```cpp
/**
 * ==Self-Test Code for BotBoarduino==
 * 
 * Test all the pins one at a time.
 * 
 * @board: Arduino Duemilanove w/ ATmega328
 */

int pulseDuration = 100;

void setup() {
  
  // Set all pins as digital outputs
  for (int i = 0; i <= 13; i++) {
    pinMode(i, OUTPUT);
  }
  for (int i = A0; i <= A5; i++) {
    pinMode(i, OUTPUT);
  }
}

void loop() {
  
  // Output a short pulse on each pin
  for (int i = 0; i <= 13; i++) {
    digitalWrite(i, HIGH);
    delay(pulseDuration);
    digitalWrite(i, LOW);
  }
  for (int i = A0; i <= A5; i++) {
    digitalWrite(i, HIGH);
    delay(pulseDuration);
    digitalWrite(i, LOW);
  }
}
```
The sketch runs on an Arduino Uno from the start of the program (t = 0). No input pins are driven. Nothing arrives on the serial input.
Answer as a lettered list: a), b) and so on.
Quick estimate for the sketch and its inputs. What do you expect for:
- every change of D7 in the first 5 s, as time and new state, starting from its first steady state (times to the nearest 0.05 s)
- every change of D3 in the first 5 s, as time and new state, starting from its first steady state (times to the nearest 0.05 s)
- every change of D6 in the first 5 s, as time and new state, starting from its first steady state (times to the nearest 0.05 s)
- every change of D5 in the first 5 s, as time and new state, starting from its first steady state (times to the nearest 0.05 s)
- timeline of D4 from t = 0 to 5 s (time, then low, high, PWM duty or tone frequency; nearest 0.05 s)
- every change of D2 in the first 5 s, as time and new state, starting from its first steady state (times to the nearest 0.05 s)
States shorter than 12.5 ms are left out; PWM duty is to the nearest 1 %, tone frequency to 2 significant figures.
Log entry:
a) 0 s low; 0.7 s high; 0.8 s low; 2.7 s high; 2.8 s low; 4.7 s high; 4.8 s low
b) 0 s low; 0.3 s high; 0.4 s low; 2.3 s high; 2.4 s low; 4.3 s high; 4.4 s low
c) 0 s low; 0.6 s high; 0.7 s low; 2.6 s high; 2.7 s low; 4.6 s high; 4.7 s low
d) 0 s low; 0.5 s high; 0.6 s low; 2.5 s high; 2.6 s low; 4.5 s high; 4.6 s low
e) 0 s low; 0.4 s high; 0.5 s low; 2.4 s high; 2.5 s low; 4.4 s high; 4.5 s low
f) 0 s low; 0.2 s high; 0.3 s low; 2.2 s high; 2.3 s low; 4.2 s high; 4.3 s low
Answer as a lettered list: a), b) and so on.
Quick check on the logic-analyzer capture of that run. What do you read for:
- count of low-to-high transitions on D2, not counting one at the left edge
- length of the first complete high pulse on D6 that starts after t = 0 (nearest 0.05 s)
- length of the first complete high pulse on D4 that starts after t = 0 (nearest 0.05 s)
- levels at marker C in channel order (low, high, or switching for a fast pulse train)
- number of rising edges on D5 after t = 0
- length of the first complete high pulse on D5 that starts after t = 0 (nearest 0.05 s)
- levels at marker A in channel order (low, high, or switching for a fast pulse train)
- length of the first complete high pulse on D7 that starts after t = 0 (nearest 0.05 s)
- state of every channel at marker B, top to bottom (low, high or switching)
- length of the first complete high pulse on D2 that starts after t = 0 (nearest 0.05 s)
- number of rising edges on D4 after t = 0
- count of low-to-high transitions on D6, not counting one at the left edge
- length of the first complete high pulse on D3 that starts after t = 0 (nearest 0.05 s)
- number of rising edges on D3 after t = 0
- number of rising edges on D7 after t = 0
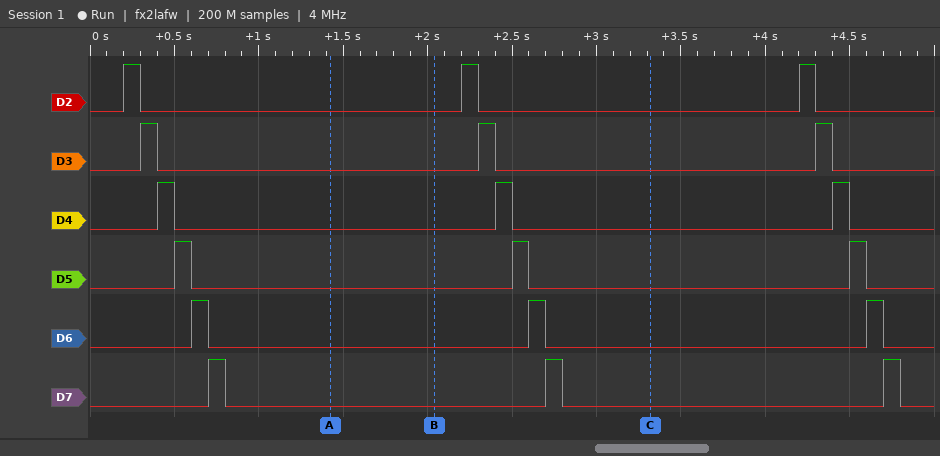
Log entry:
a) 3
b) 0.10 s
c) 0.10 s
d) D2 low, D3 low, D4 low, D5 low, D6 low, D7 low
e) 3
f) 0.10 s
g) D2 low, D3 low, D4 low, D5 low, D6 low, D7 low
h) 0.10 s
i) D2 low, D3 low, D4 low, D5 low, D6 low, D7 low
j) 0.10 s
k) 3
l) 3
m) 0.10 s
n) 3
o) 3
